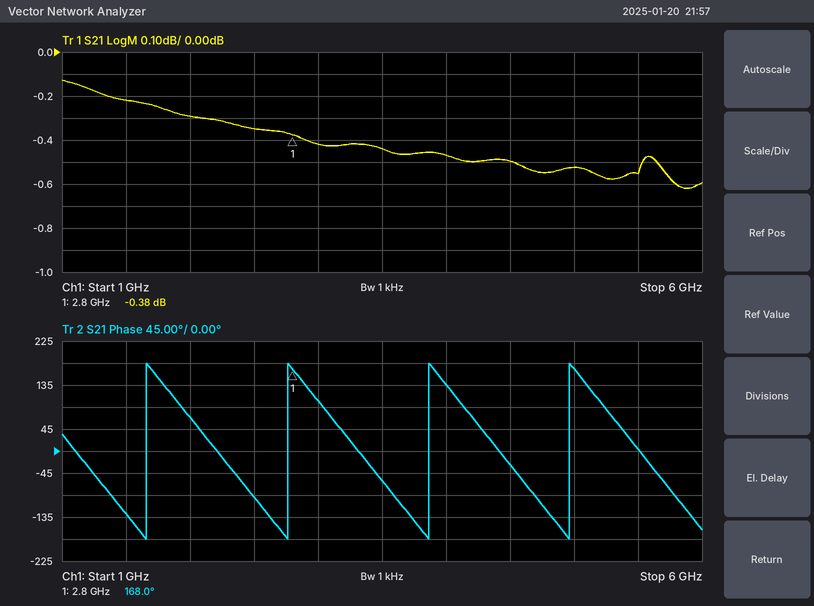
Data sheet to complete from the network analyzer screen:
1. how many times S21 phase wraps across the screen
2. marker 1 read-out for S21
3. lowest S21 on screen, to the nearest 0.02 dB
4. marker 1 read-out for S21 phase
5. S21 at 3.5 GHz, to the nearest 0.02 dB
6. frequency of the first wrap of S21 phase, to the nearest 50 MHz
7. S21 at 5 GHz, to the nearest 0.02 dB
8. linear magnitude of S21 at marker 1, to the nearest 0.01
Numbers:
4
-0.38 dB
-0.62 dB
168.0°
-0.44 dB
1.65 GHz
-0.52 dB
0.96
